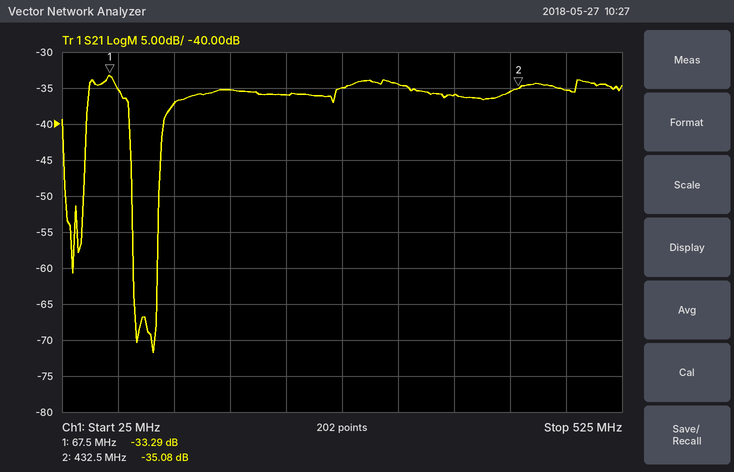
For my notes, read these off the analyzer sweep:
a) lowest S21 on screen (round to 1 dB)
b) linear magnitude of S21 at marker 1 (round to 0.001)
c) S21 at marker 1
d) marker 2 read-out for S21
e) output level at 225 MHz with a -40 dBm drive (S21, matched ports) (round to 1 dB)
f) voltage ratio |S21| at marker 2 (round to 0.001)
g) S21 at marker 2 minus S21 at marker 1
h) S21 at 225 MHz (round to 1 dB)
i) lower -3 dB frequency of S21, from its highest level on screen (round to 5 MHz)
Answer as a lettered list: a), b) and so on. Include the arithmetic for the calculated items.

a) -72 dB
b) 10^(-33.29/20) ≈ 0.022
c) -33.29 dB
d) -35.08 dB
e) -40 dBm + (-36 dB) = -76 dBm
f) 10^(-35.08/20) ≈ 0.018
g) -35.08 − (-33.29) = -1.79 dB
h) -36 dB
i) 50 MHz
